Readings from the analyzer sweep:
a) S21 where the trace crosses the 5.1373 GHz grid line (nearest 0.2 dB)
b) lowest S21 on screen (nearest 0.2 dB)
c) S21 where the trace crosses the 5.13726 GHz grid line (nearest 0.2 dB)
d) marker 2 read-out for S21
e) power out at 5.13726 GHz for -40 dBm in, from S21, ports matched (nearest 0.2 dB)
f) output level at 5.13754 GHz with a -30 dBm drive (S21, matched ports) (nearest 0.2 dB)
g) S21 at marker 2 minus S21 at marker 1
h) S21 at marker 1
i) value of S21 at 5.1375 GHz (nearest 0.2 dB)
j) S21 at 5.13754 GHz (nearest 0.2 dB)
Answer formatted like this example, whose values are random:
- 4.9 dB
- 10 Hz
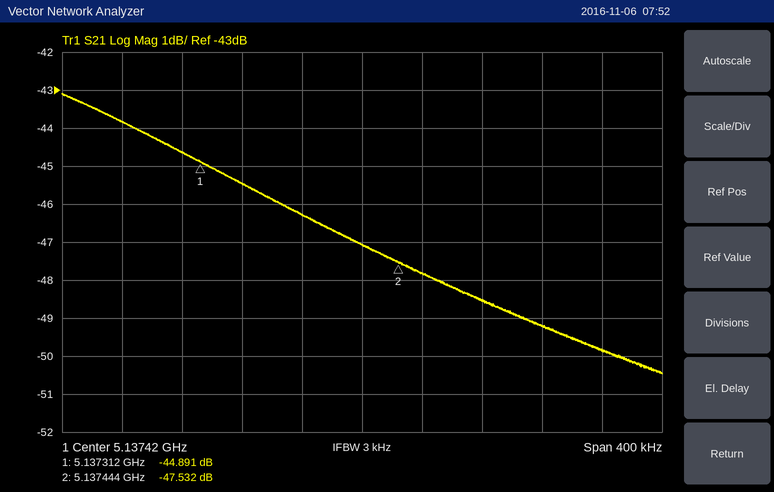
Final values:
- -44.6 dB
- -50.4 dB
- -43.8 dB
- -47.532 dB
- -83.8 dBm
- -79.2 dBm
- -2.641 dB
- -44.891 dB
- -48.6 dB
- -49.2 dB
